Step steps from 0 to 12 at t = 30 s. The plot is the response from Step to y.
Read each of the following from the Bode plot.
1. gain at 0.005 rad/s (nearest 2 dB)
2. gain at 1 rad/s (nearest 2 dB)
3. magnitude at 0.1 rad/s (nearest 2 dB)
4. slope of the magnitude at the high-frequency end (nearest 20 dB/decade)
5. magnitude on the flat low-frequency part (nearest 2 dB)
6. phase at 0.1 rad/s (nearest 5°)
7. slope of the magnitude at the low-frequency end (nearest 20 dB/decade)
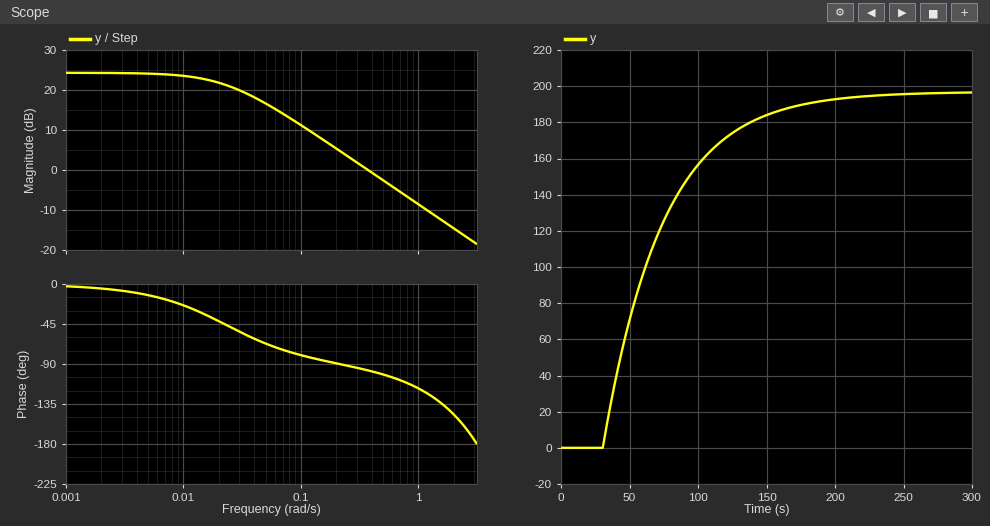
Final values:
24 dB
-8 dB
12 dB
-20 dB/decade
24 dB
-80°
0 dB/decade
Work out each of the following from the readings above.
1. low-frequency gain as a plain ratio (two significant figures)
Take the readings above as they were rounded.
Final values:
16
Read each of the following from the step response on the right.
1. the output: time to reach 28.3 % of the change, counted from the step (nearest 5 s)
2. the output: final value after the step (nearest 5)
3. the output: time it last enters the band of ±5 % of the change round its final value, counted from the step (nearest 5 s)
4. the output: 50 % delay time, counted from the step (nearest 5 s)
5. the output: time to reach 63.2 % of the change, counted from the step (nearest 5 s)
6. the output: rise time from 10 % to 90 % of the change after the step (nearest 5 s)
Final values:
15 s
195
130 s
30 s
45 s
95 s
